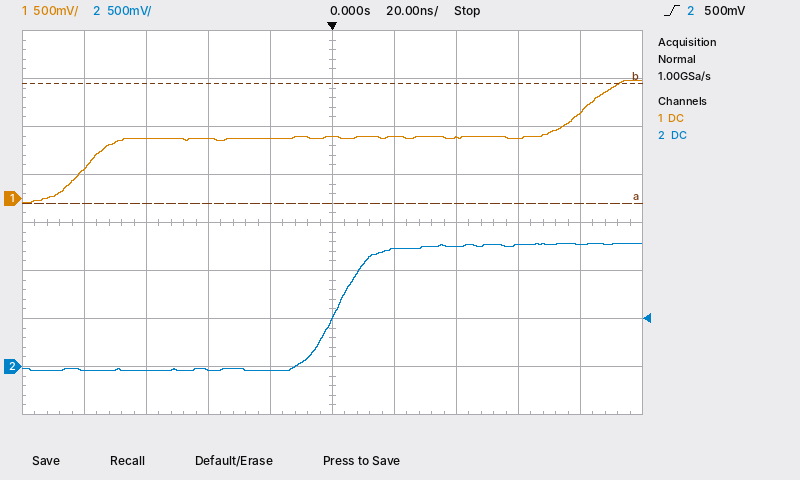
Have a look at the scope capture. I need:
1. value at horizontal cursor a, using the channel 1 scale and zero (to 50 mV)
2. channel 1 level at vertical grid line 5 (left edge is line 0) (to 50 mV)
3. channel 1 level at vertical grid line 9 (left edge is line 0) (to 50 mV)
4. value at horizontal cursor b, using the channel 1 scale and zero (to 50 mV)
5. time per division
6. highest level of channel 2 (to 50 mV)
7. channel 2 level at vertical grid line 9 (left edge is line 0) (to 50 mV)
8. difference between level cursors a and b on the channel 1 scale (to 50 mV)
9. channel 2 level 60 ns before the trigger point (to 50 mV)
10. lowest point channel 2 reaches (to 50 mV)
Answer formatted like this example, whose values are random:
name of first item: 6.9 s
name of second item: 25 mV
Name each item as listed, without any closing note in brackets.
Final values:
value at horizontal cursor a, using the channel 1 scale and zero: -50 mV
channel 1 level at vertical grid line 5 (left edge is line 0): 650 mV
channel 1 level at vertical grid line 9 (left edge is line 0): 900 mV
value at horizontal cursor b, using the channel 1 scale and zero: 1.20 V
time per division: 20 ns
highest level of channel 2: 1.30 V
channel 2 level at vertical grid line 9 (left edge is line 0): 1.25 V
difference between level cursors a and b on the channel 1 scale: 1.25 V
channel 2 level 60 ns before the trigger point: -50 mV
lowest point channel 2 reaches: -50 mV
